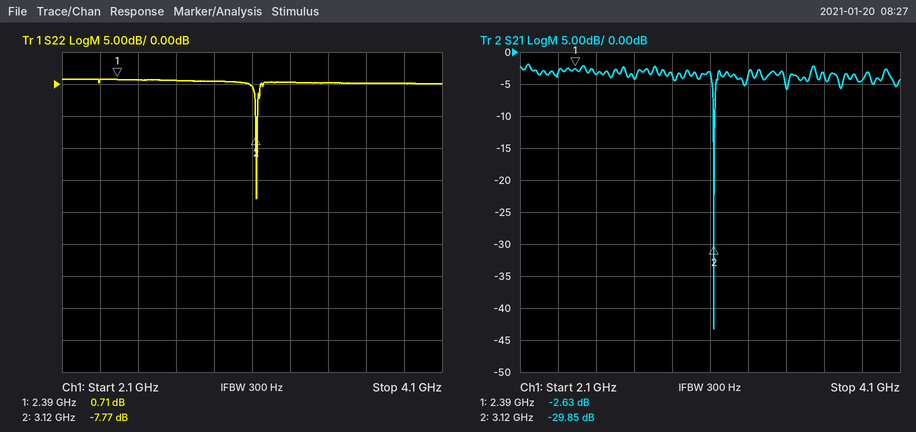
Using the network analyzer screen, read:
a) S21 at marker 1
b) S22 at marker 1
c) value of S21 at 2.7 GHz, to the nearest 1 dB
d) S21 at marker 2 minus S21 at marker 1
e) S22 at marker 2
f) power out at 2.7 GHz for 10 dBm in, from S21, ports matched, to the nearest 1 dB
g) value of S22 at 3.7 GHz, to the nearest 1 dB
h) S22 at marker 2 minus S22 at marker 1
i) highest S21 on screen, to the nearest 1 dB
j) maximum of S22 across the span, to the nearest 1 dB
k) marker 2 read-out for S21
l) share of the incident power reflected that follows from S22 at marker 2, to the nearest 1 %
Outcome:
-2.63 dB
0.71 dB
-4 dB
-27.22 dB
-7.77 dB
6 dBm
0 dB
-8.48 dB
-2 dB
1 dB
-29.85 dB
17 %
